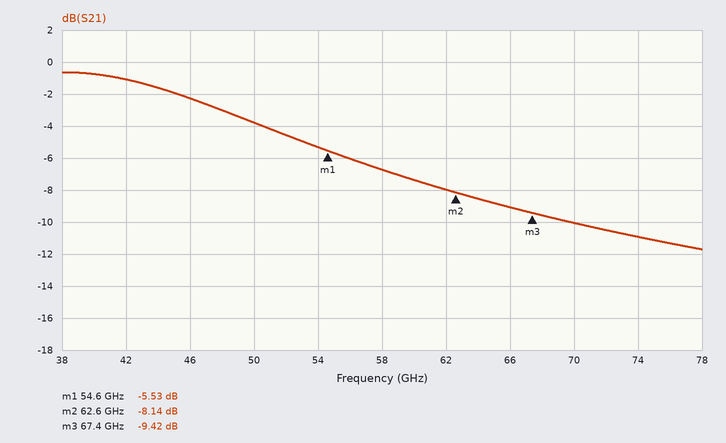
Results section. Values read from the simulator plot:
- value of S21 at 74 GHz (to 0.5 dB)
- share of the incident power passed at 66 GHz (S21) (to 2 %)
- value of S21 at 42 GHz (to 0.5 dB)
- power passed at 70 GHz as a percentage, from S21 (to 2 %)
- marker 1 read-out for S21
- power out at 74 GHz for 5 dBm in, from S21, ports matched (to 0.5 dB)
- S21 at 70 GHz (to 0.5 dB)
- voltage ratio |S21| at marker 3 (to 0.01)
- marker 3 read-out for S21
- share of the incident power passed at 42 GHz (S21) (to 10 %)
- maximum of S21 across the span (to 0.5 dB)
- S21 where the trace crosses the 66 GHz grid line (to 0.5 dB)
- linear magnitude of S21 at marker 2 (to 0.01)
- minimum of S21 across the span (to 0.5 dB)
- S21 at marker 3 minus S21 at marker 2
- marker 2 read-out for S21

-11.0 dB
12 %
-1.0 dB
10 %
-5.53 dB
-6.0 dBm
-10.0 dB
0.34
-9.42 dB
80 %
-0.5 dB
-9.0 dB
0.39
-11.5 dB
-1.28 dB
-8.14 dB
